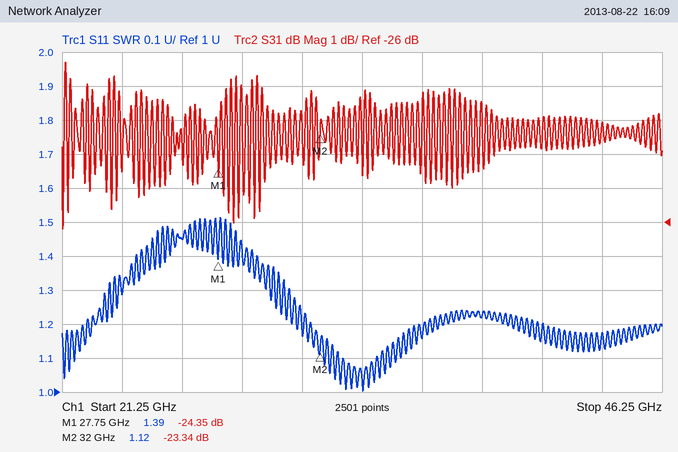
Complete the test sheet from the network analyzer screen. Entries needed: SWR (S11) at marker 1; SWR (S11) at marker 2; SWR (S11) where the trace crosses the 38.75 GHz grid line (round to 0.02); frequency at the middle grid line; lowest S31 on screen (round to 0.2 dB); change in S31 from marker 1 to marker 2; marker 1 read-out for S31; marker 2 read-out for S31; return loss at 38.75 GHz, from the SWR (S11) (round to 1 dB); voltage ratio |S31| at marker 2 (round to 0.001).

1.39
1.12
1.22
33.75 GHz
-26.2 dB
1.01 dB
-24.35 dB
-23.34 dB
20 dB
0.068
